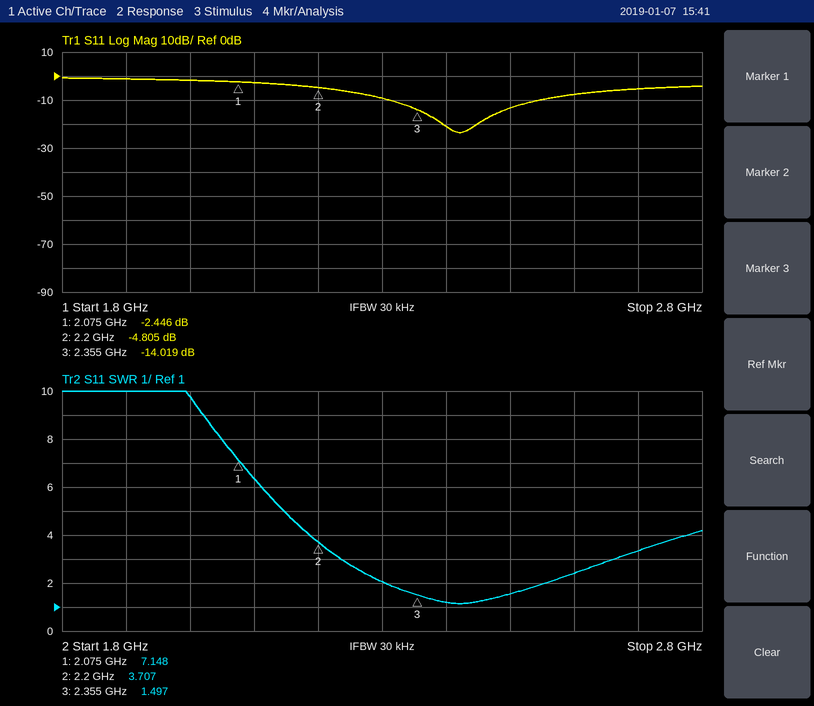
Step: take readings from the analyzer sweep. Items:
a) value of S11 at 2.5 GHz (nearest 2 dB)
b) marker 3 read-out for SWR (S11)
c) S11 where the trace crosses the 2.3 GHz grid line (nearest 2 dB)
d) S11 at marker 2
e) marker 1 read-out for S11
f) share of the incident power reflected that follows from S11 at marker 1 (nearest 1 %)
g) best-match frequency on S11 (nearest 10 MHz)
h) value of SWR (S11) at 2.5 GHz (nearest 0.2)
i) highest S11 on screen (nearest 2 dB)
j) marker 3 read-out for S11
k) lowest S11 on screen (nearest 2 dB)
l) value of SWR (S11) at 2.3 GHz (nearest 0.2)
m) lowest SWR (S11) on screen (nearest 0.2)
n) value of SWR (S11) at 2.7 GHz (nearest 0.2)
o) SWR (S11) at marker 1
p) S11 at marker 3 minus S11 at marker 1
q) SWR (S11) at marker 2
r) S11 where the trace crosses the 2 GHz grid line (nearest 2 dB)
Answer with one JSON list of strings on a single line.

["-14 dB", "1.497", "-10 dB", "-4.805 dB", "-2.446 dB", "57 %", "2.42 GHz", "1.6", "0 dB", "-14.019 dB", "-24 dB", "2.0", "1.2", "3.4", "7.148", "-11.573 dB", "3.707", "-2 dB"]
